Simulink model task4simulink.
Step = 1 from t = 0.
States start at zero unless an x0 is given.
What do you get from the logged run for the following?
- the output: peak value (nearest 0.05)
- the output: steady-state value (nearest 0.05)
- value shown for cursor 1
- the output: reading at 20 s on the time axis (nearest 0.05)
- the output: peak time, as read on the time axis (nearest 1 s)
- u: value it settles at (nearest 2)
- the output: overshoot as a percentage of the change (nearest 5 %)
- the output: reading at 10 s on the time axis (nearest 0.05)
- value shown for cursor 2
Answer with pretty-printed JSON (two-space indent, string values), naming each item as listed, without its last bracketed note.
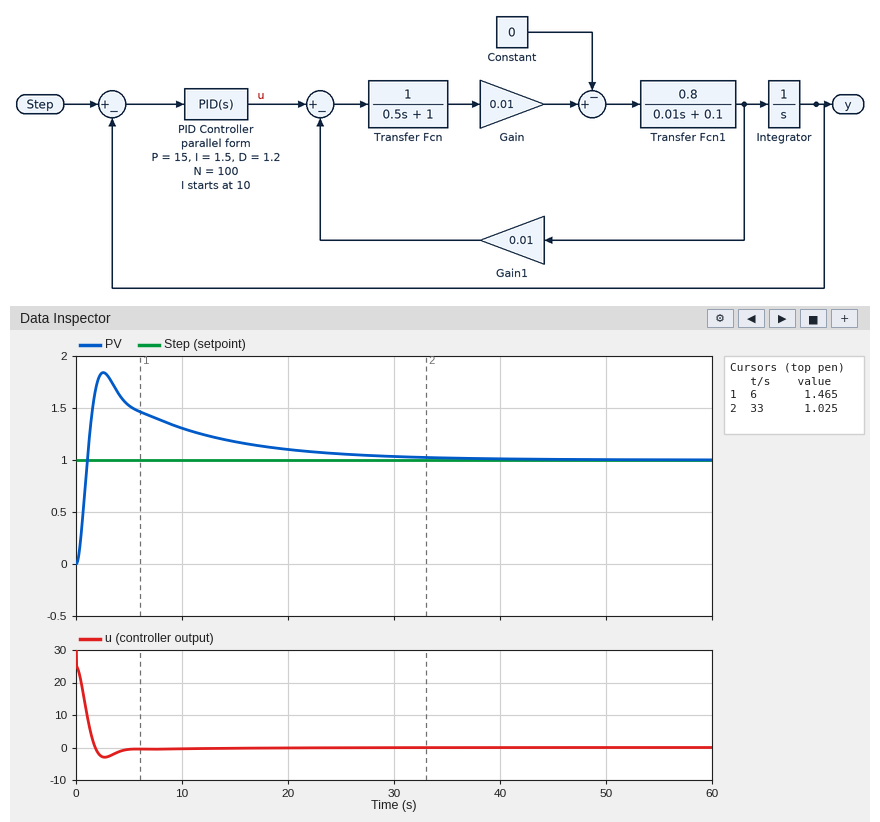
{
  "the output: peak value": "1.85",
  "the output: steady-state value": "1.00",
  "value shown for cursor 1": "1.465",
  "the output: reading at 20 s on the time axis": "1.10",
  "the output: peak time, as read on the time axis": "3 s",
  "u: value it settles at": "0",
  "the output: overshoot as a percentage of the change": "85 %",
  "the output: reading at 10 s on the time axis": "1.30",
  "value shown for cursor 2": "1.025"
}
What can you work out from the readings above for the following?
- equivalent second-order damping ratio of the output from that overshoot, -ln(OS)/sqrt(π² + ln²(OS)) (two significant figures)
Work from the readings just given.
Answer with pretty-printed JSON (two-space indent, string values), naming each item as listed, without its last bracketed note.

{
  "equivalent second-order damping ratio of the output from that overshoot, -ln(OS)/sqrt(π² + ln²(OS))": "0.052"
}
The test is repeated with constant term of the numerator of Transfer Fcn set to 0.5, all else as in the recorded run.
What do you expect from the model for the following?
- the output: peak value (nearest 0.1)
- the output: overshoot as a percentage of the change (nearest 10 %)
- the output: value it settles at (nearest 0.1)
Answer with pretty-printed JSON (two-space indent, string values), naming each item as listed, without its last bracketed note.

{
  "the output: peak value": "1.7",
  "the output: overshoot as a percentage of the change": "70 %",
  "the output: value it settles at": "1.0"
}
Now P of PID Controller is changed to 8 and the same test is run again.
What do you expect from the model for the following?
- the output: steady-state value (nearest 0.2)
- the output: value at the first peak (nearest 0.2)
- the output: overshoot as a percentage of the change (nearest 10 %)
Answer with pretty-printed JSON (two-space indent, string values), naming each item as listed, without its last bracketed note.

{
  "the output: steady-state value": "1.0",
  "the output: value at the first peak": "2.2",
  "the output: overshoot as a percentage of the change": "120 %"
}
